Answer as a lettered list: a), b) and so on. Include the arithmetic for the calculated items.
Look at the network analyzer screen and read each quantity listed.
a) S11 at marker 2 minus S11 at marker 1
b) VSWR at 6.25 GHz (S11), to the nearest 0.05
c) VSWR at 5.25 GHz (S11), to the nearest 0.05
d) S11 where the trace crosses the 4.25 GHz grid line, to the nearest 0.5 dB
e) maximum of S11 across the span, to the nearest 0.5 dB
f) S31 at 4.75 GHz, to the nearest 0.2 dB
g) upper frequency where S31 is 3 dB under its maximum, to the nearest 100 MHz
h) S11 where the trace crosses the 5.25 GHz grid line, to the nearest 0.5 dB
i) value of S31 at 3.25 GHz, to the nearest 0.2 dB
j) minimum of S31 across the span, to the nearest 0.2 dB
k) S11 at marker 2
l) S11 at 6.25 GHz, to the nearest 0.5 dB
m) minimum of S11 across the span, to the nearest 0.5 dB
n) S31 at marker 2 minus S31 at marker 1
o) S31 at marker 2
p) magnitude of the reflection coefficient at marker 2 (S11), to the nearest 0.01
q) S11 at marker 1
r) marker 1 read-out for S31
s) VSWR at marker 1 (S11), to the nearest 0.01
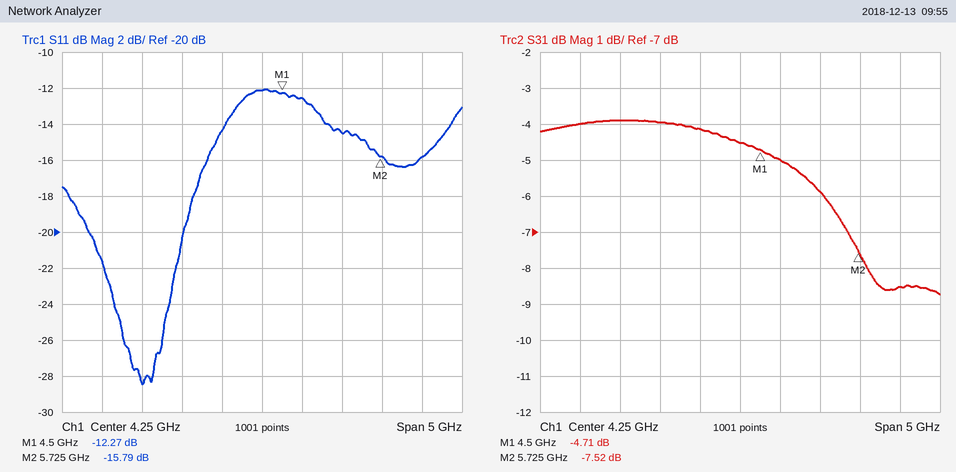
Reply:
a) -15.79 − (-12.27) = -3.52 dB
b) |Γ| = 10^(-16/20) = 0.1585; VSWR = (1 + 0.1585)/(1 − 0.1585) ≈ 1.38, so 1.40 to the nearest 0.05
c) |Γ| = 10^(-14.5/20) = 0.1884; VSWR = (1 + 0.1884)/(1 − 0.1884) ≈ 1.46, so 1.45 to the nearest 0.05
d) -12.0 dB
e) -12.0 dB
f) -5.0 dB
g) 5.6 GHz
h) -14.5 dB
i) -4.0 dB
j) -8.8 dB
k) -15.79 dB
l) -16.0 dB
m) -28.5 dB
n) -7.52 − (-4.71) = -2.81 dB
o) -7.52 dB
p) 10^(-15.79/20) ≈ 0.16
q) -12.27 dB
r) -4.71 dB
s) (1 + 0.2435)/(1 − 0.2435) ≈ 1.64
